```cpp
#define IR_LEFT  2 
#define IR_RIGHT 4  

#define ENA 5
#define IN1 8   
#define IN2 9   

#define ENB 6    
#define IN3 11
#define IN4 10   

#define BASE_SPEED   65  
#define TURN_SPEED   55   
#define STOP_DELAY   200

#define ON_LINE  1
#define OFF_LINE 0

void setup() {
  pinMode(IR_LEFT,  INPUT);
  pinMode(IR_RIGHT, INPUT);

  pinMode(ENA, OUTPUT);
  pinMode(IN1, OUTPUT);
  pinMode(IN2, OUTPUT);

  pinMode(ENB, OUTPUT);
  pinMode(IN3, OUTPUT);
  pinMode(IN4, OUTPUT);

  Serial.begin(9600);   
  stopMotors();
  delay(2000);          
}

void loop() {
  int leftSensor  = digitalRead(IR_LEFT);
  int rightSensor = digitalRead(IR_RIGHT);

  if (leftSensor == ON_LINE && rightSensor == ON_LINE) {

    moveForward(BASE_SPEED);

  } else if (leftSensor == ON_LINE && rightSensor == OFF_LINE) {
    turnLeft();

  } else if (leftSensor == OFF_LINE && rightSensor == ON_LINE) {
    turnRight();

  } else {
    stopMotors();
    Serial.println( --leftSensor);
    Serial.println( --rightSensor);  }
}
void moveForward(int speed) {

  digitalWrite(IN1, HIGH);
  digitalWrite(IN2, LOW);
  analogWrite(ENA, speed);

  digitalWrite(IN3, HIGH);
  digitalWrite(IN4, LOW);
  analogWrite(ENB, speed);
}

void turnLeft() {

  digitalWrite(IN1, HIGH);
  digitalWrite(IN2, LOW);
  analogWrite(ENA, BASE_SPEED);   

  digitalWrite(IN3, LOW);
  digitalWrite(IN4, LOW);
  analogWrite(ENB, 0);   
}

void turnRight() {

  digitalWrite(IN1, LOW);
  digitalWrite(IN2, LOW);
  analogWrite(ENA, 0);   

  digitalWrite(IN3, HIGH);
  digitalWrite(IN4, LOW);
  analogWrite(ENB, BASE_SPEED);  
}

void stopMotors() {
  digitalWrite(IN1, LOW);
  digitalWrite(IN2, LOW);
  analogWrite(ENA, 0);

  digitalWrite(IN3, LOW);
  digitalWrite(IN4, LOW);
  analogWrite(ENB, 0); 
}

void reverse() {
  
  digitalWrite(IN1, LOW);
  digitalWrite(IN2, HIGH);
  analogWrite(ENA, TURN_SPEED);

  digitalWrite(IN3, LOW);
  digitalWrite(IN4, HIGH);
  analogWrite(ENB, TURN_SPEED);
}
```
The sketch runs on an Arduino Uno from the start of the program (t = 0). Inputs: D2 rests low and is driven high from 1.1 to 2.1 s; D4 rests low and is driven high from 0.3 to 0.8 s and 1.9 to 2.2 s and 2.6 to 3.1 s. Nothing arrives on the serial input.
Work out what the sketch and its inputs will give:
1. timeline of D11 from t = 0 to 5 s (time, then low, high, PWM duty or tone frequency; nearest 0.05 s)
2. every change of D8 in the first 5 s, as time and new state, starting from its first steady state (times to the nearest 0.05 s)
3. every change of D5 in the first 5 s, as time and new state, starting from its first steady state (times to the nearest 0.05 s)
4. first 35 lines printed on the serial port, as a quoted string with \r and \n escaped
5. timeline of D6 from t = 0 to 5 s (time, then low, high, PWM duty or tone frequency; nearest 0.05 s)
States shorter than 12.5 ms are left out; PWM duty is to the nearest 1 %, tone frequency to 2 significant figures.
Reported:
0 s low; 2 s high; 2.2 s low; 2.6 s high; 3.1 s low
0 s low; 2 s high; 2.1 s low
0 s low; 2 s PWM 26 %; 2.1 s low
"-1\r\n-1\r\n-1\r\n-1\r\n-1\r\n-1\r\n-1\r\n-1\r\n-1\r\n-1\r\n-1\r\n-1\r\n-1\r\n-1\r\n-1\r\n-1\r\n-1\r\n-1\r\n-1\r\n-1\r\n-1\r\n-1\r\n-1\r\n-1\r\n-1\r\n-1\r\n-1\r\n-1\r\n-1\r\n-1\r\n-1\r\n-1\r\n-1\r\n-1\r\n-1\r\n"
0 s low; 2 s PWM 26 %; 2.2 s low; 2.6 s PWM 26 %; 3.1 s low
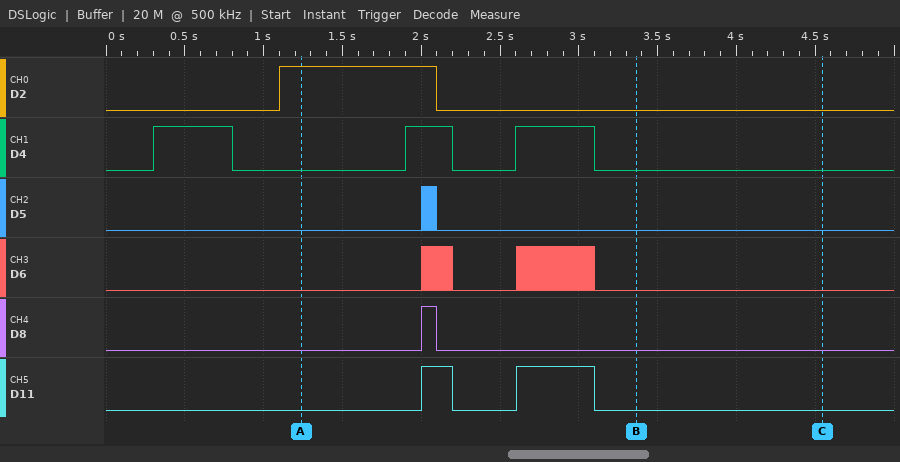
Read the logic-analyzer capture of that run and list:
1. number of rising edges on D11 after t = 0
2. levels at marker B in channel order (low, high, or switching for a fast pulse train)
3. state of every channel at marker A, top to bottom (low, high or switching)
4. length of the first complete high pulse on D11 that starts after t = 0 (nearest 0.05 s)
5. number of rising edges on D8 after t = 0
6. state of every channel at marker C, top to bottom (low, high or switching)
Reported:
2
D2 low, D4 low, D5 low, D6 low, D8 low, D11 low
D2 high, D4 low, D5 low, D6 low, D8 low, D11 low
0.20 s
1
D2 low, D4 low, D5 low, D6 low, D8 low, D11 low
